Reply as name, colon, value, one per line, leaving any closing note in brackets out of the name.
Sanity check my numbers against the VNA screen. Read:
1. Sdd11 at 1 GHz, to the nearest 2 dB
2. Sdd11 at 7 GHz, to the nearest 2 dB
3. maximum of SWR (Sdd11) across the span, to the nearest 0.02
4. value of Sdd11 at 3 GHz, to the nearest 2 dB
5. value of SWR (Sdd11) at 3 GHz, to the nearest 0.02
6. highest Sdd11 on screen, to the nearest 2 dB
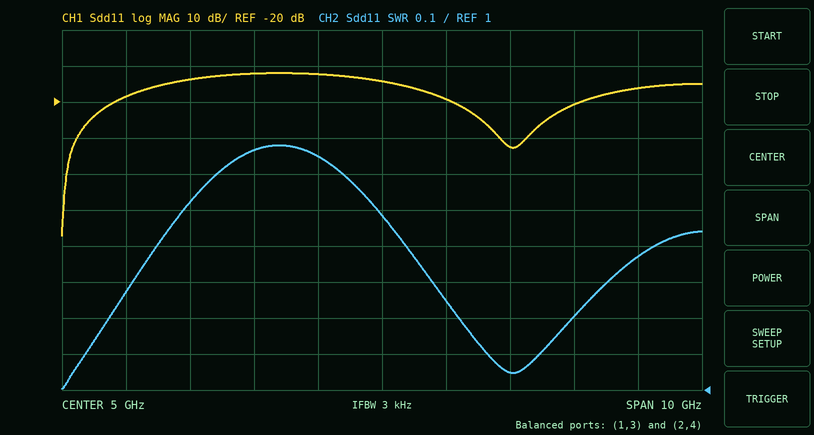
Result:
Sdd11 at 1 GHz, to the nearest 2 dB: -18 dB
Sdd11 at 7 GHz, to the nearest 2 dB: -32 dB
maximum of SWR (Sdd11) across the span, to the nearest 0.02: 1.68
value of Sdd11 at 3 GHz, to the nearest 2 dB: -12 dB
value of SWR (Sdd11) at 3 GHz, to the nearest 0.02: 1.66
highest Sdd11 on screen, to the nearest 2 dB: -12 dB
